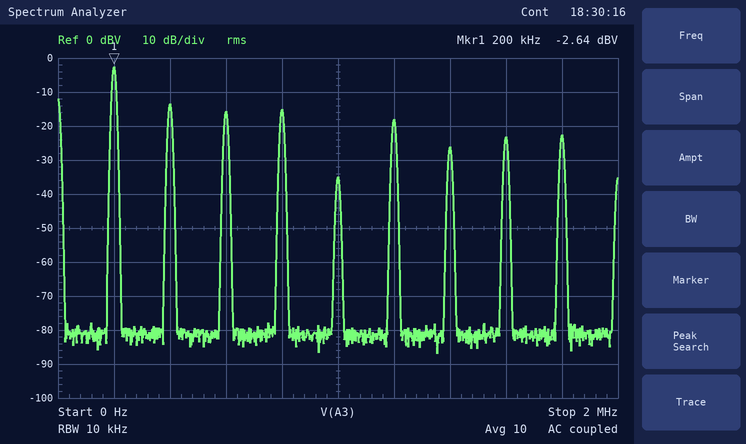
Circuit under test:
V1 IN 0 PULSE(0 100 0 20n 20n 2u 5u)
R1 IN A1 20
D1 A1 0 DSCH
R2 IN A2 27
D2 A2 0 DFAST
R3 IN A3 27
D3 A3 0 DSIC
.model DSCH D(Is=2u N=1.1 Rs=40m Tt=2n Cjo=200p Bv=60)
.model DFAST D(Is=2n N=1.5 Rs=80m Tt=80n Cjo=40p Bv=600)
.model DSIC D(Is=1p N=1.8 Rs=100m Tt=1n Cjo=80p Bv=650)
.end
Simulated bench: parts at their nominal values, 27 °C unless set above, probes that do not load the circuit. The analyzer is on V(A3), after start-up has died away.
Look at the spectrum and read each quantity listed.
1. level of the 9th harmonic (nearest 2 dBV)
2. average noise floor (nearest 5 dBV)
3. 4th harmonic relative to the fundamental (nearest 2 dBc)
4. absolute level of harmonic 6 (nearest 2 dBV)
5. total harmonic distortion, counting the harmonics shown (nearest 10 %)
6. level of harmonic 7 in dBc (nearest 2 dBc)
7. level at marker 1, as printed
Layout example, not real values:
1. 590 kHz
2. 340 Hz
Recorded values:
1. -22 dBV
2. -80 dBV
3. -12 dBc
4. -18 dBV
5. 50 %
6. -24 dBc
7. -2.64 dBV
